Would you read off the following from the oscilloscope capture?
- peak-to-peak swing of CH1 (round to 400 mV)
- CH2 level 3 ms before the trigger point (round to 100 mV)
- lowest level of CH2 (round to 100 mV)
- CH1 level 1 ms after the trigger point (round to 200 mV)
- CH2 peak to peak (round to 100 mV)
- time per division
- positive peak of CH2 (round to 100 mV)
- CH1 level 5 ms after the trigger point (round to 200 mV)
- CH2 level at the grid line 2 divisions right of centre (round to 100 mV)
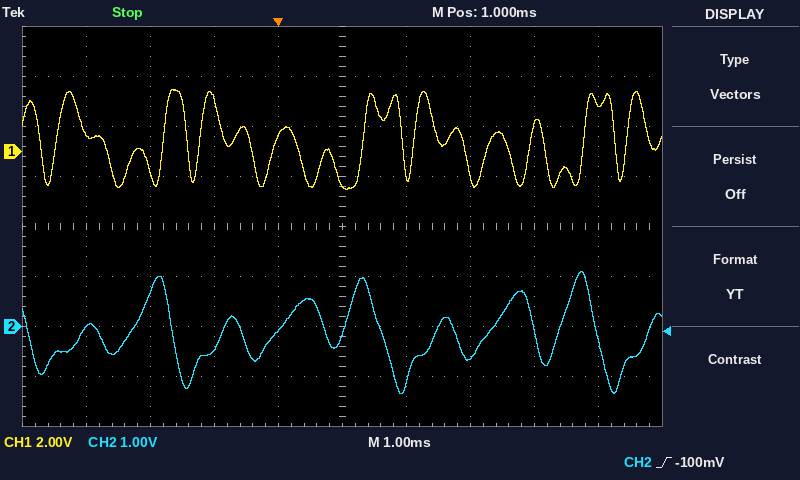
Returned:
4.0 V
0.0 V
-1.3 V
-1.4 V
2.4 V
1 ms
1.1 V
2.0 V
-600 mV
